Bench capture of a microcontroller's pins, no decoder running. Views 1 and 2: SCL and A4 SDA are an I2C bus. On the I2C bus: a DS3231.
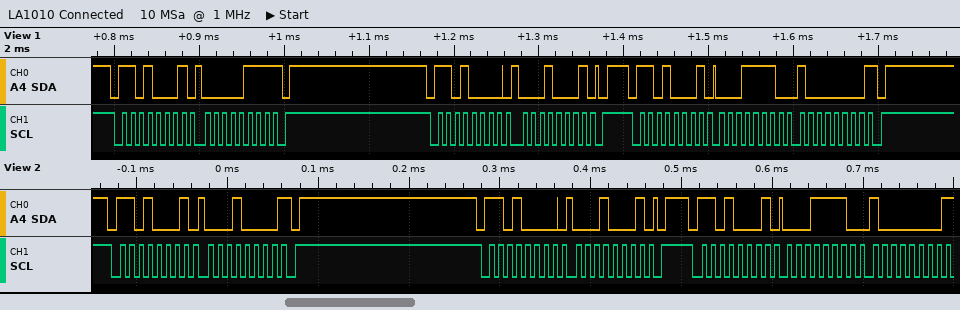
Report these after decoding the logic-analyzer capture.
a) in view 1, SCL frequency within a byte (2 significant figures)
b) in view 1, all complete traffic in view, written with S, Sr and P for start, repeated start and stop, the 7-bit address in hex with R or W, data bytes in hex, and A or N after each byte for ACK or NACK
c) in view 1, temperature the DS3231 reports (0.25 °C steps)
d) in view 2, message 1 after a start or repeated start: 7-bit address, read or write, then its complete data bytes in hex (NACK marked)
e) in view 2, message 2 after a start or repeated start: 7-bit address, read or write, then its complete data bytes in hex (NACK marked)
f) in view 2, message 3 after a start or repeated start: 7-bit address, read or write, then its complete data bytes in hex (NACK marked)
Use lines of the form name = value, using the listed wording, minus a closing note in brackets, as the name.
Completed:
in view 1, SCL frequency within a byte = 100 kHz
in view 1, all complete traffic in view, written with S, Sr and P for start, repeated start and stop, the 7-bit address in hex with R or W, data bytes in hex, and A or N after each byte for ACK or NACK = S 68R A 07 N P S 68W A 11 A P S 68R A 1E A 80 N P
in view 1, temperature the DS3231 reports = 30.50 °C
in view 2, message 1 after a start or repeated start: 7-bit address, read or write, then its complete data bytes in hex = 0x68 read: 10 NACK
in view 2, message 2 after a start or repeated start: 7-bit address, read or write, then its complete data bytes in hex = 0x68 write: 11
in view 2, message 3 after a start or repeated start: 7-bit address, read or write, then its complete data bytes in hex = 0x68 read: 1E 80 NACK
